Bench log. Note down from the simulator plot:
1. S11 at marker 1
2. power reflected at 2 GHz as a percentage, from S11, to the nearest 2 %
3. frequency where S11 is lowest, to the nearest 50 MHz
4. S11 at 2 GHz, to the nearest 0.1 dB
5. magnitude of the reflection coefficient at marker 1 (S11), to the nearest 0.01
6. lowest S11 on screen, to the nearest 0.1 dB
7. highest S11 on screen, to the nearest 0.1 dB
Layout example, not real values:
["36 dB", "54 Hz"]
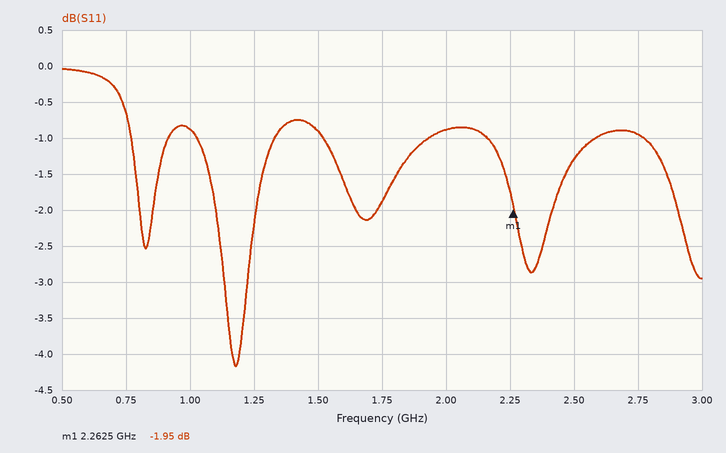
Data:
["-1.95 dB", "82 %", "1.20 GHz", "-0.9 dB", "0.80", "-4.2 dB", "0.0 dB"]
